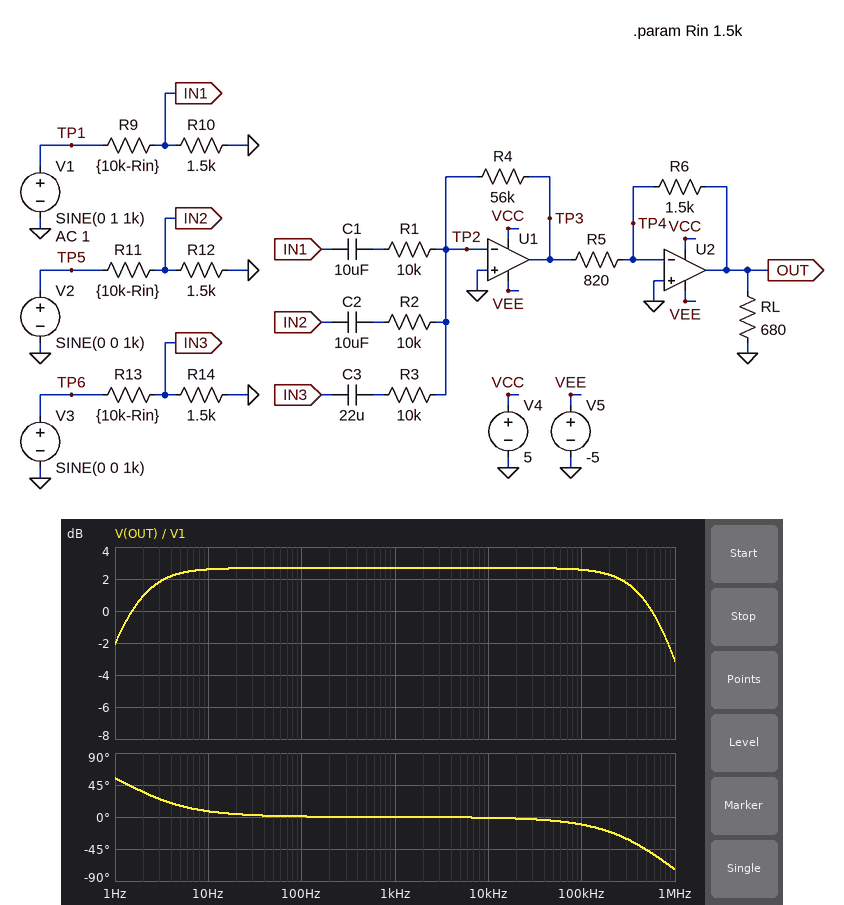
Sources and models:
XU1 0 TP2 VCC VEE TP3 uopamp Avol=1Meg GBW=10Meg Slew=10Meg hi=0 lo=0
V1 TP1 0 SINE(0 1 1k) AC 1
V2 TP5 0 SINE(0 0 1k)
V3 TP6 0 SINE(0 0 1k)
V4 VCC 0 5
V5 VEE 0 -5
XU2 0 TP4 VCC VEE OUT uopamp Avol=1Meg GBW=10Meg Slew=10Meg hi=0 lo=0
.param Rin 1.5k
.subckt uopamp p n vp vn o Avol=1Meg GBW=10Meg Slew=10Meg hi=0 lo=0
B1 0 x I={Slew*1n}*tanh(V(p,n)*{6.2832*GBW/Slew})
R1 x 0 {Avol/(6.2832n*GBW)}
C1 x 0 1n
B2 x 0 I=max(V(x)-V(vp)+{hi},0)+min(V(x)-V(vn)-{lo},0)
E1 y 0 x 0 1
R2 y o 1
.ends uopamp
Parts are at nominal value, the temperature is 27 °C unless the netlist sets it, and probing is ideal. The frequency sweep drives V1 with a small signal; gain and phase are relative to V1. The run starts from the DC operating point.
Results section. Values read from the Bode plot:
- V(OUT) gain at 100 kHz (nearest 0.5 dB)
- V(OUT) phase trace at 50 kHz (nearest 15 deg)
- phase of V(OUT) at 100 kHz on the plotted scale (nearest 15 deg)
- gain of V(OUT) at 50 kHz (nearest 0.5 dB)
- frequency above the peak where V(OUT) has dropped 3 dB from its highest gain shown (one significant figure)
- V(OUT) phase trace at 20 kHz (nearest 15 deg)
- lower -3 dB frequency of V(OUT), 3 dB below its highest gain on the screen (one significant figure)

2.5 dB
0 deg
-15 deg
2.5 dB
600 kHz
0 deg
1 Hz
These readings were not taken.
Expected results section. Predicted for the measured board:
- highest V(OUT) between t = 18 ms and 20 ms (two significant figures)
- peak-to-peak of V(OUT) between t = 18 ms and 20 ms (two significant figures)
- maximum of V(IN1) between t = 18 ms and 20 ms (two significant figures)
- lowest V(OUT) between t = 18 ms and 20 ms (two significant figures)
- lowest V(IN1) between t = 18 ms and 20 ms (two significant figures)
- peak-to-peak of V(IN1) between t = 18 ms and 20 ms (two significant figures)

1.4 V
2.7 V
130 mV
-1.4 V
-130 mV
270 mV
